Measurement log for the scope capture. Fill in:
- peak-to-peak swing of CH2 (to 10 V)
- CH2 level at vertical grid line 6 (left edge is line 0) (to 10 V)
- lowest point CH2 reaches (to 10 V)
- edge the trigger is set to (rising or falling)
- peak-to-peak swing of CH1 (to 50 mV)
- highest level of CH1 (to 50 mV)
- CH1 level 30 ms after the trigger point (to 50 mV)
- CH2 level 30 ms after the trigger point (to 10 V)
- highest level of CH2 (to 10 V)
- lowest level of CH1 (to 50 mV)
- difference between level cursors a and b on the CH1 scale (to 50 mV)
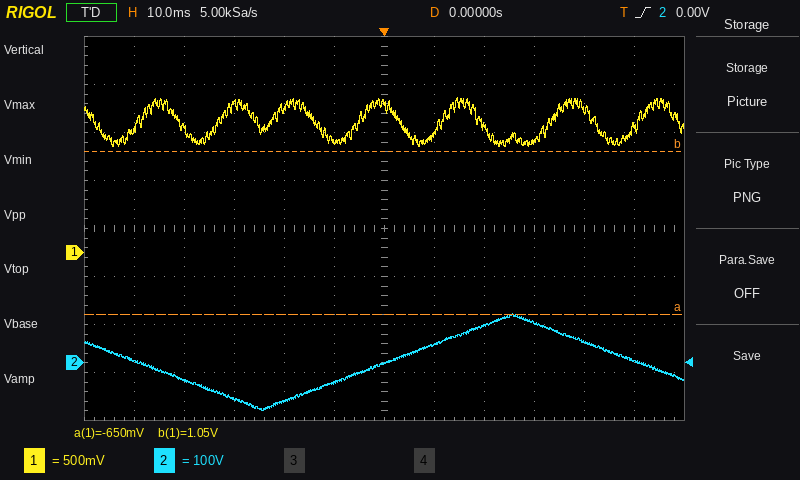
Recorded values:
200 V
0 V
-100 V
rising
500 mV
1.60 V
1.15 V
80 V
100 V
1.10 V
1.70 V
